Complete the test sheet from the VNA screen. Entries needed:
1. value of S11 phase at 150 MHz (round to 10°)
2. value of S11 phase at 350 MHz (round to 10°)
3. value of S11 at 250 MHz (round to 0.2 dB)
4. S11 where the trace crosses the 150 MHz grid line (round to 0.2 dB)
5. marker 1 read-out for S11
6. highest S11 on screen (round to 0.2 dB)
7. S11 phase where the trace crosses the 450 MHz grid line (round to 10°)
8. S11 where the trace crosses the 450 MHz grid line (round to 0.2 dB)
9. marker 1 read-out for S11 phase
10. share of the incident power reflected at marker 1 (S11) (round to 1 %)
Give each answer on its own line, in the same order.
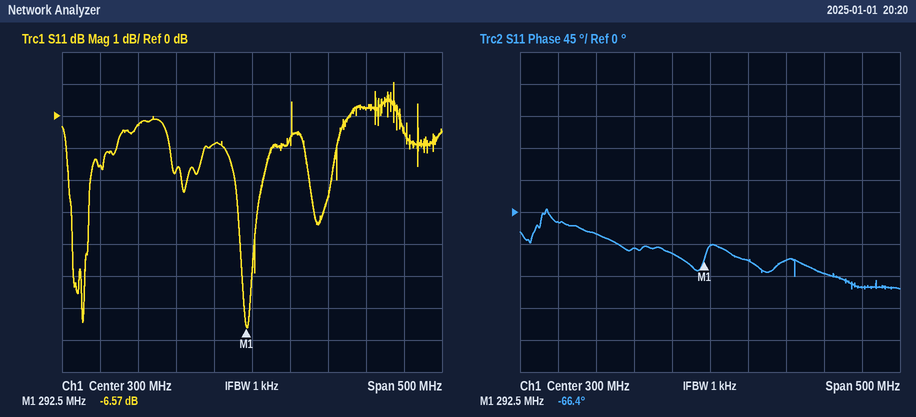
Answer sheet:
-30°
-70°
-0.8 dB
-0.2 dB
-6.57 dB
1.0 dB
-90°
0.2 dB
-66.4°
22 %
